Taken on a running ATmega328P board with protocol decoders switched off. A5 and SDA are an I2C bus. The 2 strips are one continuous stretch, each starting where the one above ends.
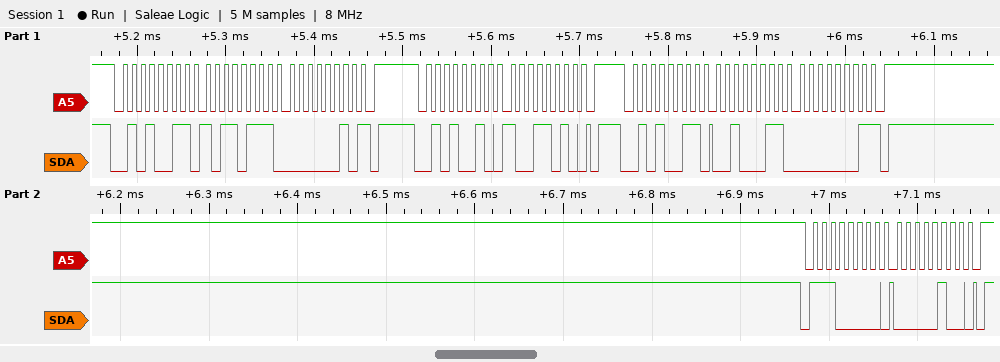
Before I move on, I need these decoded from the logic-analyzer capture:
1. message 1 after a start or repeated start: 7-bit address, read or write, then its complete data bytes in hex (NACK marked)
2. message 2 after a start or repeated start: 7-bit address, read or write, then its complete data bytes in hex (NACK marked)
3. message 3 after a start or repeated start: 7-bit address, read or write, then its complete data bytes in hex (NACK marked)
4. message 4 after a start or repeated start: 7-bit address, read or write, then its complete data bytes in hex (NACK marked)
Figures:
0x29 read: B7 02 NACK
0x29 write: 9A
0x29 read: 23 01 NACK
0x70 write: 04
